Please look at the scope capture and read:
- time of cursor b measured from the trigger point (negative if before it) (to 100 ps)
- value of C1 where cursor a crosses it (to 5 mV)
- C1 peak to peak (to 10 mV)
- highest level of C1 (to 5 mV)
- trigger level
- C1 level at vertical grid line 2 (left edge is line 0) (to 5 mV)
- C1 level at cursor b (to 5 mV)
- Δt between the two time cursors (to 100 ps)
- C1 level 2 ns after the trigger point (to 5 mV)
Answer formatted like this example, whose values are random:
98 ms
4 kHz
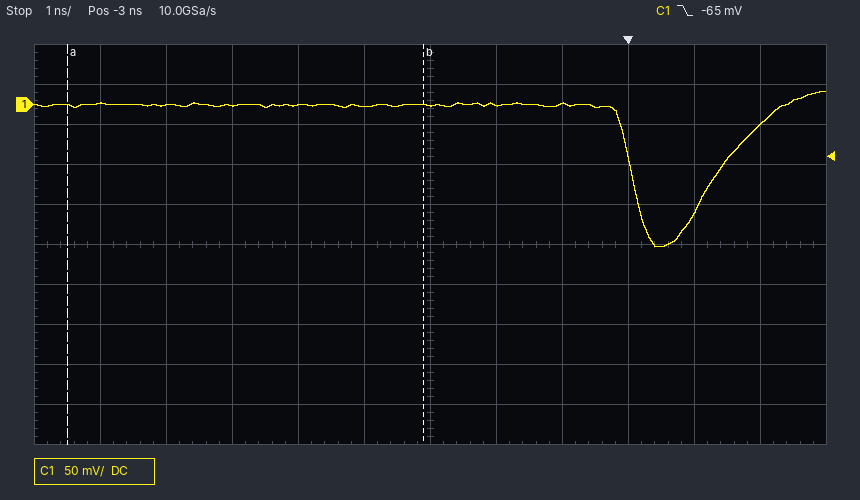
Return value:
-3.1 ns
0 mV
190 mV
15 mV
-65 mV
0 mV
0 mV
5.4 ns
-25 mV
